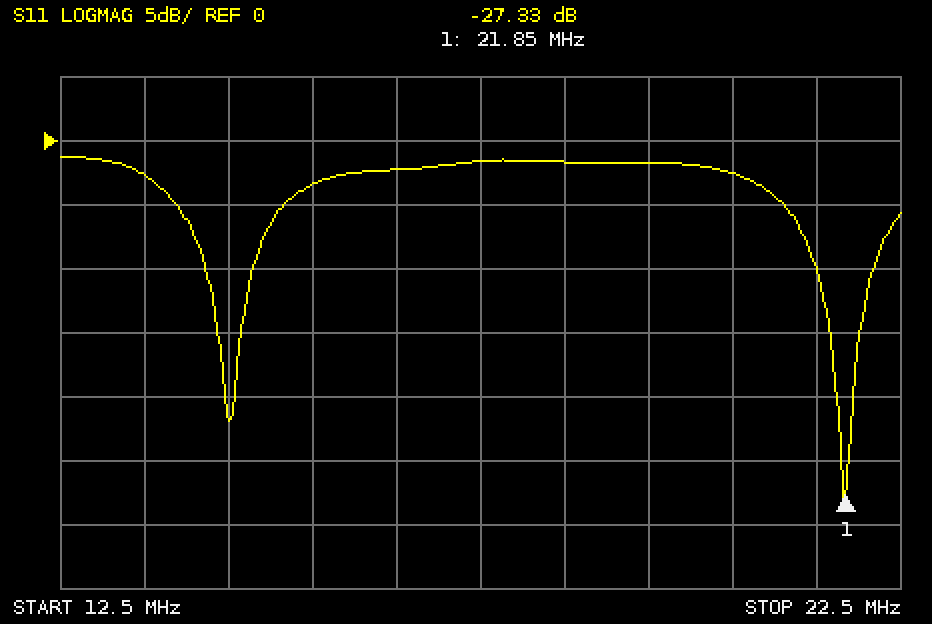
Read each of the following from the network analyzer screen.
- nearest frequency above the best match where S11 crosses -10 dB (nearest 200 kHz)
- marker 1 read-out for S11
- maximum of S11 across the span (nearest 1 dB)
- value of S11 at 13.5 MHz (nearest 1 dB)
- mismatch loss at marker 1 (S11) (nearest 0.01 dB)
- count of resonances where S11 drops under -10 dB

22.2 MHz
-27.33 dB
-1 dB
-3 dB
0.01 dB
2
